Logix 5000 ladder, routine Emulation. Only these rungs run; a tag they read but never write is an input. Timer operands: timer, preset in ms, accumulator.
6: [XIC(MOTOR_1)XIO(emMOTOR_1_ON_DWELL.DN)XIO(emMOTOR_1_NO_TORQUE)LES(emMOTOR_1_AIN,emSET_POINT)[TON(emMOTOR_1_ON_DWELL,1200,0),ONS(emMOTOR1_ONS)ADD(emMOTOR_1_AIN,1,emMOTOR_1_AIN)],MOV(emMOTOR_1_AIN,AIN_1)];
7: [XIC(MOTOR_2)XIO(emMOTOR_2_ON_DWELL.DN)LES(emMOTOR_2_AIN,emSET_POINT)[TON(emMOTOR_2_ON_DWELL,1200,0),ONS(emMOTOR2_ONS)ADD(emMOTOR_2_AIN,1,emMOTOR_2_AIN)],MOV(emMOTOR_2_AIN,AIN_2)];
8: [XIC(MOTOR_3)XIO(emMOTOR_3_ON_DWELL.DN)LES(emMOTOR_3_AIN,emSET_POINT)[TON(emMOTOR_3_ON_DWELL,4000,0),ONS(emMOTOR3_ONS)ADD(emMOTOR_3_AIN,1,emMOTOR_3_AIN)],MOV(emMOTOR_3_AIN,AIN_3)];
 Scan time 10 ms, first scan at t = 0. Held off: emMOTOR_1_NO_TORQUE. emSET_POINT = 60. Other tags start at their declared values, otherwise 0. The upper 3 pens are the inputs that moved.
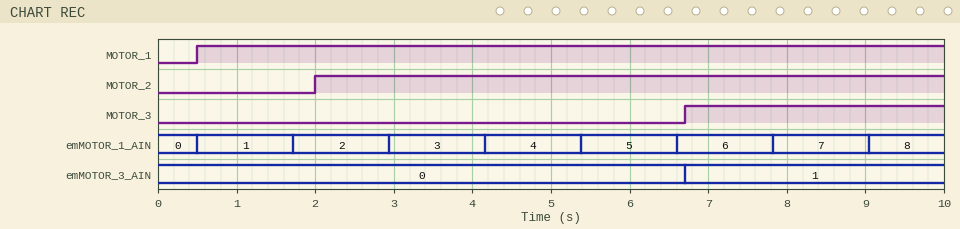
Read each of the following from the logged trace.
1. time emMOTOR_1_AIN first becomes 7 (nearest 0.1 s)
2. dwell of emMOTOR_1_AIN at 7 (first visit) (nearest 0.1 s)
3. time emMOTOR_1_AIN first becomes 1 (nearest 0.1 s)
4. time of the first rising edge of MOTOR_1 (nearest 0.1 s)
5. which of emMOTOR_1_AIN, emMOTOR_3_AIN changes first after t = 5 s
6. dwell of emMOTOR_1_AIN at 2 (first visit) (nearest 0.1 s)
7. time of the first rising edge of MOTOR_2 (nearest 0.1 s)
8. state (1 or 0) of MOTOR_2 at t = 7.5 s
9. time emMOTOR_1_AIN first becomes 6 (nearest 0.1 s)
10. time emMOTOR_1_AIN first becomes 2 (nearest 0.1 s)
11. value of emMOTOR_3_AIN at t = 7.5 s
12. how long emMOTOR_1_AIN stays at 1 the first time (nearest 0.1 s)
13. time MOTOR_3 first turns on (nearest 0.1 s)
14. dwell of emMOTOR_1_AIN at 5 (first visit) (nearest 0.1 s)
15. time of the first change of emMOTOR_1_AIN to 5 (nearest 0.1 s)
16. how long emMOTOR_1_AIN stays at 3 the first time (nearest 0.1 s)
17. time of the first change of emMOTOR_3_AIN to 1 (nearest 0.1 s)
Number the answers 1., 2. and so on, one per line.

1. 7.8 s
2. 1.2 s
3. 0.5 s
4. 0.5 s
5. emMOTOR_1_AIN
6. 1.2 s
7. 2.0 s
8. 1
9. 6.6 s
10. 1.7 s
11. 1
12. 1.2 s
13. 6.7 s
14. 1.2 s
15. 5.4 s
16. 1.2 s
17. 6.7 s
